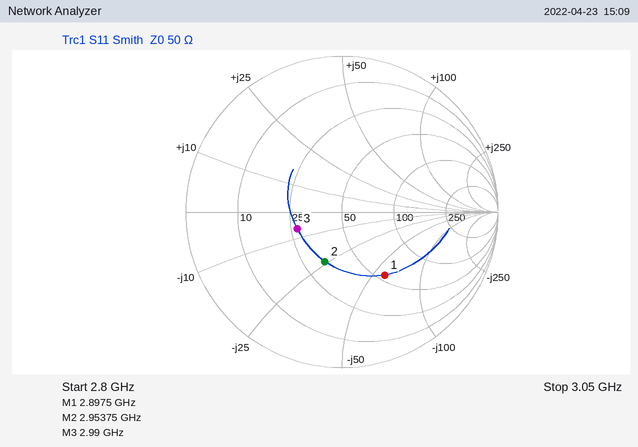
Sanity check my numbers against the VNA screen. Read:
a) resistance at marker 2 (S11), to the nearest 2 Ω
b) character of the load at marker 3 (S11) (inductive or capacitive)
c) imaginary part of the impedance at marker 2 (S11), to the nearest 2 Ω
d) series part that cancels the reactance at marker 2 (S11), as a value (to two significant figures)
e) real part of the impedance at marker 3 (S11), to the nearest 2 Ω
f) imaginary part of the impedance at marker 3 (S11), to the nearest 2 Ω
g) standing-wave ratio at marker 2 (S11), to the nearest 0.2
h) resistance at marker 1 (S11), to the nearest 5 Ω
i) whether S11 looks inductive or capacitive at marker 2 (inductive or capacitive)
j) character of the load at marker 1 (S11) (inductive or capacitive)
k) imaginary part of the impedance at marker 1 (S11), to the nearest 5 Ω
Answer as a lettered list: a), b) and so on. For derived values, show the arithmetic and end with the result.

a) 34 Ω
b) capacitive
c) -24 Ω
d) L = 24 Ω/(2π × 2.95375 GHz) ≈ 1.3 nH
e) 28 Ω
f) -6 Ω
g) 2.0
h) 55 Ω
i) capacitive
j) capacitive
k) -60 Ω
